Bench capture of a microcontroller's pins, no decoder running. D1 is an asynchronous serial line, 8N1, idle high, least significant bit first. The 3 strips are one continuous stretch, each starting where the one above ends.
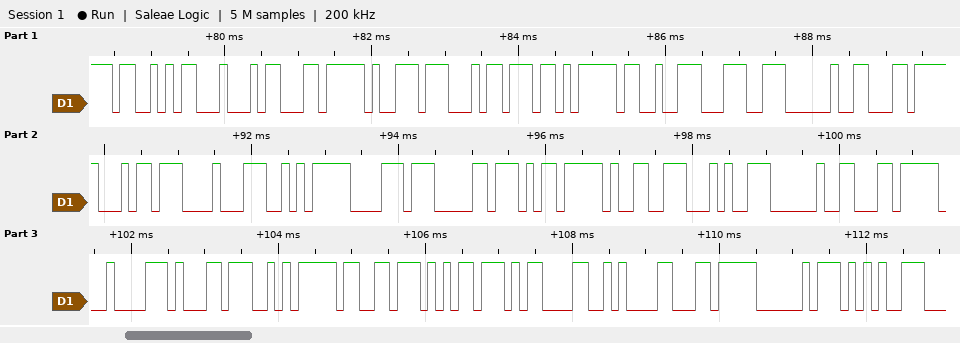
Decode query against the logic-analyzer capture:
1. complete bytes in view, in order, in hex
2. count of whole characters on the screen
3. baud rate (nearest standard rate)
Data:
0x53 0x44 0xEC 0xB9 0xB4 0xEB 0x93 0x9C 0x20 0xEC 0xB4 0x88 0xEA 0xB8 0xB0 0xED 0x99 0x94 0x20 0xEC 0x84 0xB1 0xEA 0xB3 0xB5 0x0D 0x0A 0xEC 0xA0 0x95
30
9600 baud
